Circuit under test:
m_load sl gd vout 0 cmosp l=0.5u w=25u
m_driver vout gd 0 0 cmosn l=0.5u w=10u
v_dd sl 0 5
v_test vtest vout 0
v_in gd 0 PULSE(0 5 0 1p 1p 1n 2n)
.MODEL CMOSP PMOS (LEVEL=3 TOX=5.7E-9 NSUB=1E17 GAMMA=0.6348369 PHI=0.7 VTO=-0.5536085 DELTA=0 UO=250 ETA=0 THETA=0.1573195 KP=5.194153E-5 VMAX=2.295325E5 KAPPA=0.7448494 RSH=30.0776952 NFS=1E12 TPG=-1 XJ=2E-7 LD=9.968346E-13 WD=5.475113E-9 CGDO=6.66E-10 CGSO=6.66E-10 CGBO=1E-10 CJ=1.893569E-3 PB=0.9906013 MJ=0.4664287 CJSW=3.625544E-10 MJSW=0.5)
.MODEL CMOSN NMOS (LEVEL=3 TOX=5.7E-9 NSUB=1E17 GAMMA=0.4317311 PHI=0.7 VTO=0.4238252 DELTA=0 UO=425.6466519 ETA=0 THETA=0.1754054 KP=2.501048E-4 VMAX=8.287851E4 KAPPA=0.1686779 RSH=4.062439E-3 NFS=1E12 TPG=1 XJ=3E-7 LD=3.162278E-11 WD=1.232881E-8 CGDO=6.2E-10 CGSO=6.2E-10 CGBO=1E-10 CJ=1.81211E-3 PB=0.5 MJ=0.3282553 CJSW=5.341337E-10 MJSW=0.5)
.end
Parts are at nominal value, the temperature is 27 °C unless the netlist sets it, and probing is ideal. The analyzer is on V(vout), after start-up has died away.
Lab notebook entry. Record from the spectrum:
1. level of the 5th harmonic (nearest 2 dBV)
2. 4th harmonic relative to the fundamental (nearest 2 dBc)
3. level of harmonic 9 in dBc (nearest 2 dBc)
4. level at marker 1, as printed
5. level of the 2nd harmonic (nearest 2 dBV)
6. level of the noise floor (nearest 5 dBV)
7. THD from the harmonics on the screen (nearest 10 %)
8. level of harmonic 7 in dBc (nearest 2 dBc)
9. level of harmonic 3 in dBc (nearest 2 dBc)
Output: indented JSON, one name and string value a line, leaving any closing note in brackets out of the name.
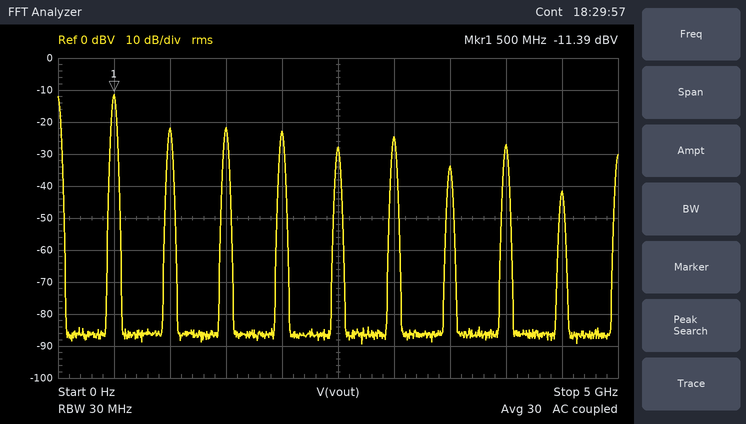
{
  "level of the 5th harmonic": "-28 dBV",
  "4th harmonic relative to the fundamental": "-12 dBc",
  "level of harmonic 9 in dBc": "-30 dBc",
  "level at marker 1, as printed": "-11.39 dBV",
  "level of the 2nd harmonic": "-22 dBV",
  "level of the noise floor": "-85 dBV",
  "THD from the harmonics on the screen": "60 %",
  "level of harmonic 7 in dBc": "-22 dBc",
  "level of harmonic 3 in dBc": "-10 dBc"
}
